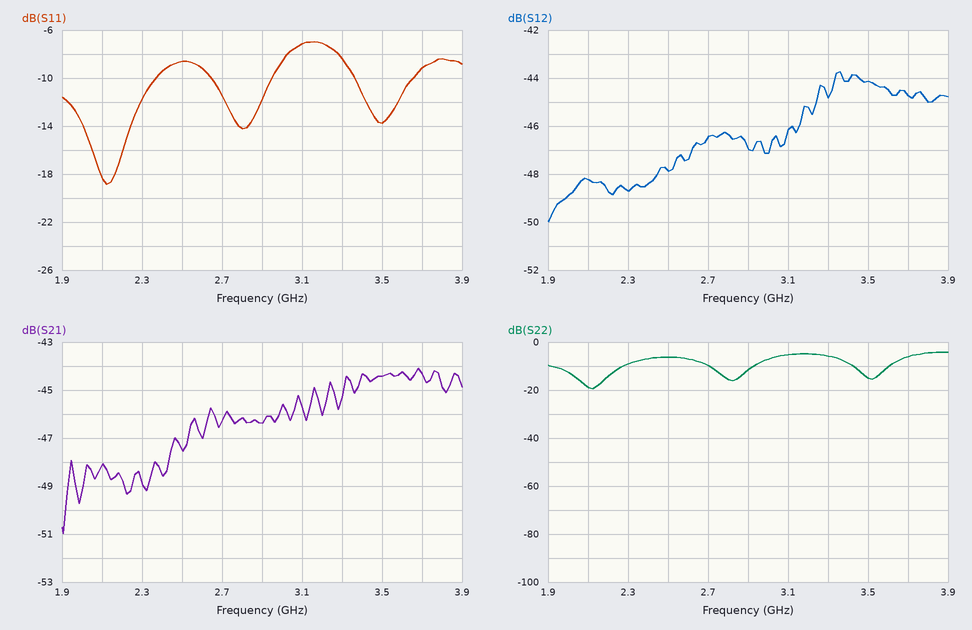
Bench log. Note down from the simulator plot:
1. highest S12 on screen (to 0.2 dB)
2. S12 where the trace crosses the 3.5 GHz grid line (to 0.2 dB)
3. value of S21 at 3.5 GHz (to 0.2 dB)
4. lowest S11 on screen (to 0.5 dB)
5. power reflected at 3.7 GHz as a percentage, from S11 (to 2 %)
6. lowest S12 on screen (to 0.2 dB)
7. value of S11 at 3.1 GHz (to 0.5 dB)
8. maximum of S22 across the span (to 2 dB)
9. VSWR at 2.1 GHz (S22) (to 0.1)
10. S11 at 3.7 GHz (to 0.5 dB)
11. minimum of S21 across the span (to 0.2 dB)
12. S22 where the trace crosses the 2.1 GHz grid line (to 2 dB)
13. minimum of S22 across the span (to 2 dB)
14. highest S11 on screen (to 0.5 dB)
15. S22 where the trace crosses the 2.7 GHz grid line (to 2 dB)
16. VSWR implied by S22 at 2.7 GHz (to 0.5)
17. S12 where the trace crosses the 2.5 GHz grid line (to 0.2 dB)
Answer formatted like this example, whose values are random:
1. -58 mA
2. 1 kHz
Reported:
1. -43.8 dB
2. -44.2 dB
3. -44.4 dB
4. -19.0 dB
5. 12 %
6. -50.0 dB
7. -7.0 dB
8. -4 dB
9. 1.3
10. -9.0 dB
11. -51.0 dB
12. -18 dB
13. -20 dB
14. -7.0 dB
15. -10 dB
16. 2.0
17. -47.8 dB
